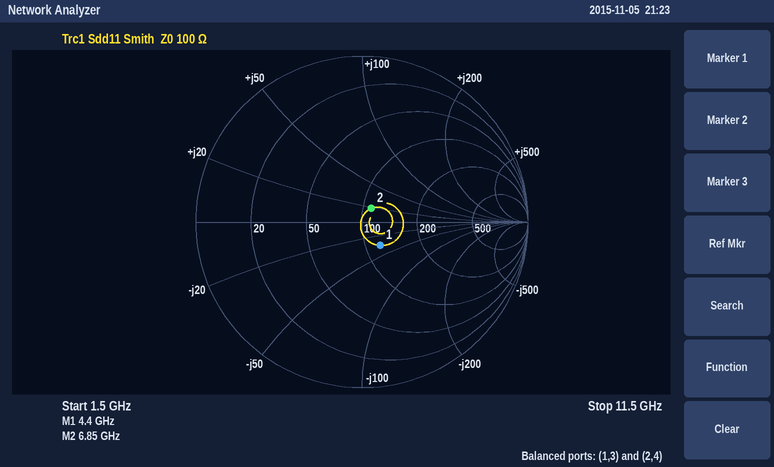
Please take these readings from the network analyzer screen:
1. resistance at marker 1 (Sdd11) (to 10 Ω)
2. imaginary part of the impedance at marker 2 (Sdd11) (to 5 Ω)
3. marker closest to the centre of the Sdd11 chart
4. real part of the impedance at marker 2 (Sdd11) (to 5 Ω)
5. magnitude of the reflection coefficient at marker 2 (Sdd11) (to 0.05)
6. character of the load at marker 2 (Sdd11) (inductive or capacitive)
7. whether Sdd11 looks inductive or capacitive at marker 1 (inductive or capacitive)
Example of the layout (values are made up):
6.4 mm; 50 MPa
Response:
120 Ω; +20 Ω; marker 2; 110 Ω; 0.10; inductive; capacitive
